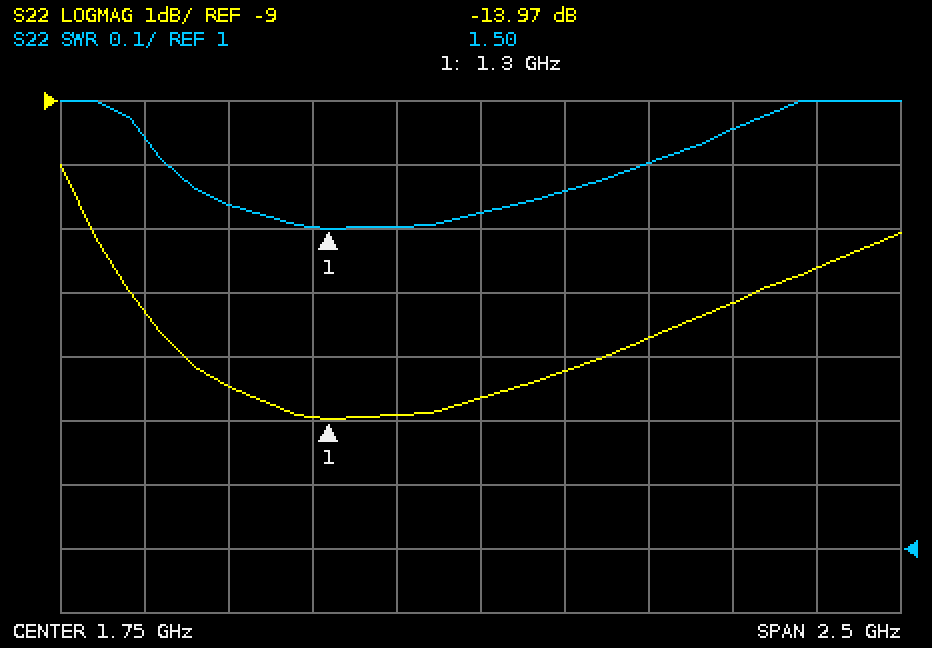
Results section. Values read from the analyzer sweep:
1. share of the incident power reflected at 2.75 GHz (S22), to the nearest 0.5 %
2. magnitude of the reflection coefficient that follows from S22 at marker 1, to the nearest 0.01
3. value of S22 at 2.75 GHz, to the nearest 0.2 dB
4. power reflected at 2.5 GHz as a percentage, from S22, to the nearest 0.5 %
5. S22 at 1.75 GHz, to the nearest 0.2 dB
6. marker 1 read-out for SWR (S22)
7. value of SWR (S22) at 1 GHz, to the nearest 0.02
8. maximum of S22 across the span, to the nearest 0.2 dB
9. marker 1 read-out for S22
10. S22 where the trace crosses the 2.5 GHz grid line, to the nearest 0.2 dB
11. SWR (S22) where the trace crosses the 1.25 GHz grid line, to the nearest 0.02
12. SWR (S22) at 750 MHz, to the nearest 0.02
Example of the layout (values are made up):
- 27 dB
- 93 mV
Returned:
- 7.0 %
- 0.20
- -11.6 dB
- 6.0 %
- -13.6 dB
- 1.50
- 1.54
- -10.0 dB
- -13.97 dB
- -12.2 dB
- 1.50
- 1.64
